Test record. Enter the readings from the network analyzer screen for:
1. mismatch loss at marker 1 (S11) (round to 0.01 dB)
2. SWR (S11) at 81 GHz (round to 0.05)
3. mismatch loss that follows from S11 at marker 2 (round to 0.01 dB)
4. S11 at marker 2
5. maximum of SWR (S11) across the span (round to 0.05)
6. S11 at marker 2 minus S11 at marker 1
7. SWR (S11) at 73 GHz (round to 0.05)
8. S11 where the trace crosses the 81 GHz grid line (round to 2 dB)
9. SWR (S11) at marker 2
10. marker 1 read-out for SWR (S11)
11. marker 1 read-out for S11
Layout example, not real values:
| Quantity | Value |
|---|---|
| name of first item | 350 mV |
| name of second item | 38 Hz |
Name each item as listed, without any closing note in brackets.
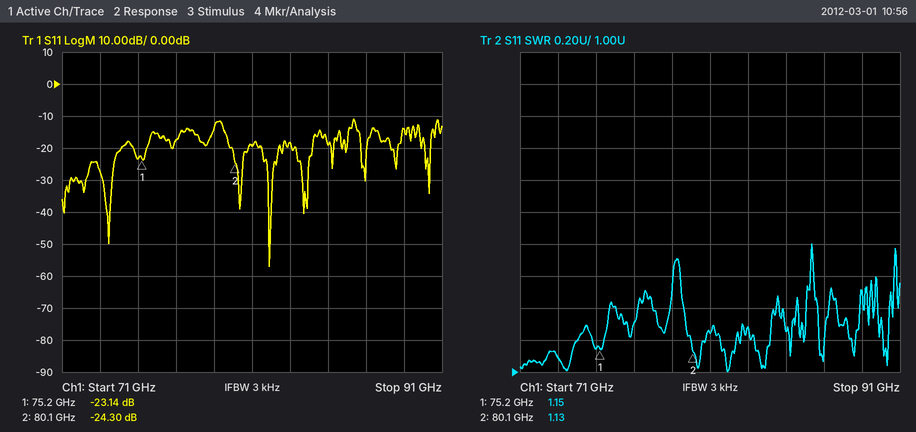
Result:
| Quantity | Value |
|---|---|
| mismatch loss at marker 1 (S11) | 0.02 dB |
| SWR (S11) at 81 GHz | 1.25 |
| mismatch loss that follows from S11 at marker 2 | 0.02 dB |
| S11 at marker 2 | -24.30 dB |
| maximum of SWR (S11) across the span | 1.80 |
| S11 at marker 2 minus S11 at marker 1 | -1.16 dB |
| SWR (S11) at 73 GHz | 1.10 |
| S11 where the trace crosses the 81 GHz grid line | -20 dB |
| SWR (S11) at marker 2 | 1.13 |
| marker 1 read-out for SWR | 1.15 |
| marker 1 read-out for S11 | -23.14 dB |
